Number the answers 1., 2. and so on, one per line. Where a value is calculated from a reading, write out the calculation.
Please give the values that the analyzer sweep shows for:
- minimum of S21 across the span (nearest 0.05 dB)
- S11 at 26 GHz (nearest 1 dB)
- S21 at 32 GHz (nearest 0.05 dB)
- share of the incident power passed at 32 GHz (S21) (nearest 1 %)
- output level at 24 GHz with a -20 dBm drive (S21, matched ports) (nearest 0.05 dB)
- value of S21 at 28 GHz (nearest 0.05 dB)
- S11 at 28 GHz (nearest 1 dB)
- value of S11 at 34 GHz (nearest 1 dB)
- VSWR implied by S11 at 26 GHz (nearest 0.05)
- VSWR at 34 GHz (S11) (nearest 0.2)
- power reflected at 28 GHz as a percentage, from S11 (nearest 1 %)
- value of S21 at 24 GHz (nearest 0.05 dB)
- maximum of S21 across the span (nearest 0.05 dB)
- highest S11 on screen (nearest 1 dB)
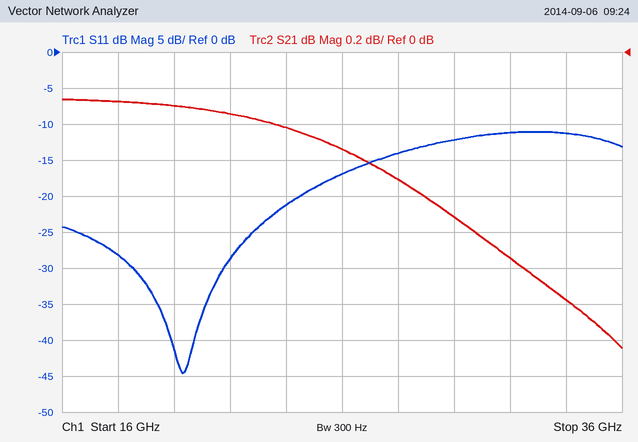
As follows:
1. -1.65 dB
2. -17 dB
3. -1.15 dB
4. 10^(-1.15/10) ≈ 77 %
5. -20 dBm + (-0.40 dB) = -20.40 dBm
6. -0.70 dB
7. -14 dB
8. -11 dB
9. |Γ| = 10^(-17/20) = 0.1413; VSWR = (1 + 0.1413)/(1 − 0.1413) ≈ 1.33, so 1.35 to the nearest 0.05
10. |Γ| = 10^(-11/20) = 0.2818; VSWR = (1 + 0.2818)/(1 − 0.2818) ≈ 1.8
11. 10^(-14/10) ≈ 4 %
12. -0.40 dB
13. -0.25 dB
14. -11 dB
